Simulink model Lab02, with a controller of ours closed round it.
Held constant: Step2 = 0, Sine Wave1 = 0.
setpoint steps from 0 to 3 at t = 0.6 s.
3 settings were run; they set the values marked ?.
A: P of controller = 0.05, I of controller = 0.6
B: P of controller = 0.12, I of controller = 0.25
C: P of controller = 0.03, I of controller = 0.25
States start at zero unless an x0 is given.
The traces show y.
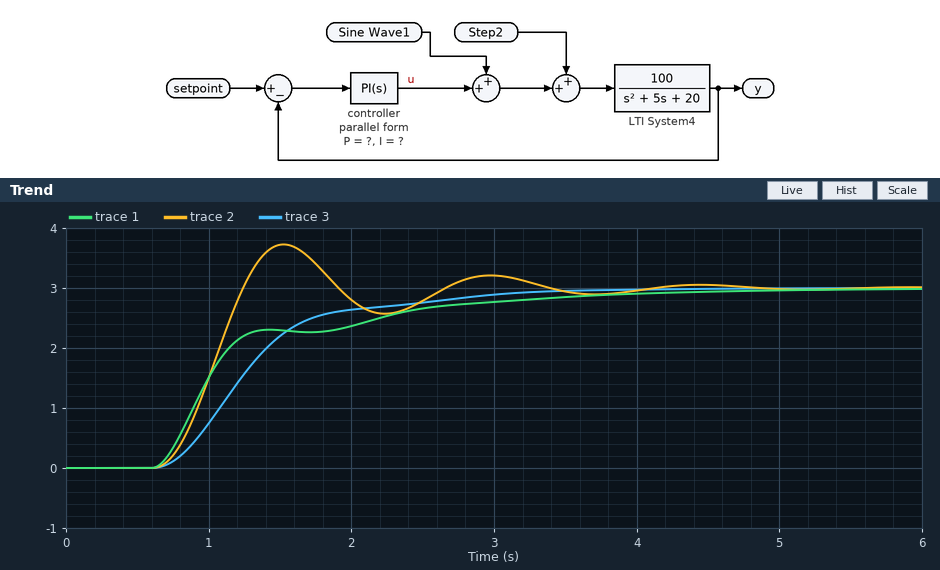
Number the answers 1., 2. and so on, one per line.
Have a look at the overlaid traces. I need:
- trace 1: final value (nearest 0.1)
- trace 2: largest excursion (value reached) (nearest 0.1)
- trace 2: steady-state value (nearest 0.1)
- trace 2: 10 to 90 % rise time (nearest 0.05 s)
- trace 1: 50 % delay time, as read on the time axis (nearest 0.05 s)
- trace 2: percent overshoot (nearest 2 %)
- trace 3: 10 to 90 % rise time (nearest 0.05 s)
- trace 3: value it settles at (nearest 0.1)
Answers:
1. 3.0
2. 3.7
3. 3.0
4. 0.40 s
5. 1.00 s
6. 24 %
7. 1.45 s
8. 3.0
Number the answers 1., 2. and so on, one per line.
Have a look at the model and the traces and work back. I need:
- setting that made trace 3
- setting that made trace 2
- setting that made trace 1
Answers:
1. C
2. A
3. B
